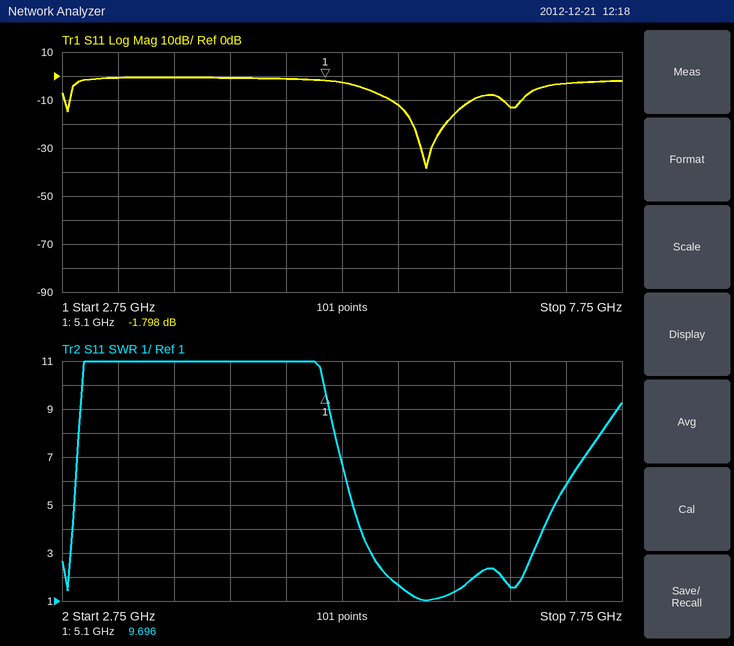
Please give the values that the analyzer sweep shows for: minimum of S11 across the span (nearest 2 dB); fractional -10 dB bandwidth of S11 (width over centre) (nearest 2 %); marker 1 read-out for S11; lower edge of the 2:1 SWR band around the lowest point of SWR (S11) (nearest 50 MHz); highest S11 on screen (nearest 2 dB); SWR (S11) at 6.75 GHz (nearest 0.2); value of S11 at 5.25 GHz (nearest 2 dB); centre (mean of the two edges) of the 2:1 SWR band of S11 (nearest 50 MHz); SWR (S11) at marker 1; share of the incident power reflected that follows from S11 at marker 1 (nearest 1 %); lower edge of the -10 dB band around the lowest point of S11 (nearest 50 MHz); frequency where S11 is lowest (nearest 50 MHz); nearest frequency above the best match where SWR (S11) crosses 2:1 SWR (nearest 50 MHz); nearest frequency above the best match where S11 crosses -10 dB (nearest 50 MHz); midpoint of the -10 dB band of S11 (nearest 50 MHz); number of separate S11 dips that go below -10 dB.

-38 dB
12 %
-1.798 dB
5.65 GHz
0 dB
1.6
-2 dB
6.05 GHz
9.696
66 %
5.70 GHz
6.00 GHz
6.45 GHz
6.40 GHz
6.05 GHz
3
